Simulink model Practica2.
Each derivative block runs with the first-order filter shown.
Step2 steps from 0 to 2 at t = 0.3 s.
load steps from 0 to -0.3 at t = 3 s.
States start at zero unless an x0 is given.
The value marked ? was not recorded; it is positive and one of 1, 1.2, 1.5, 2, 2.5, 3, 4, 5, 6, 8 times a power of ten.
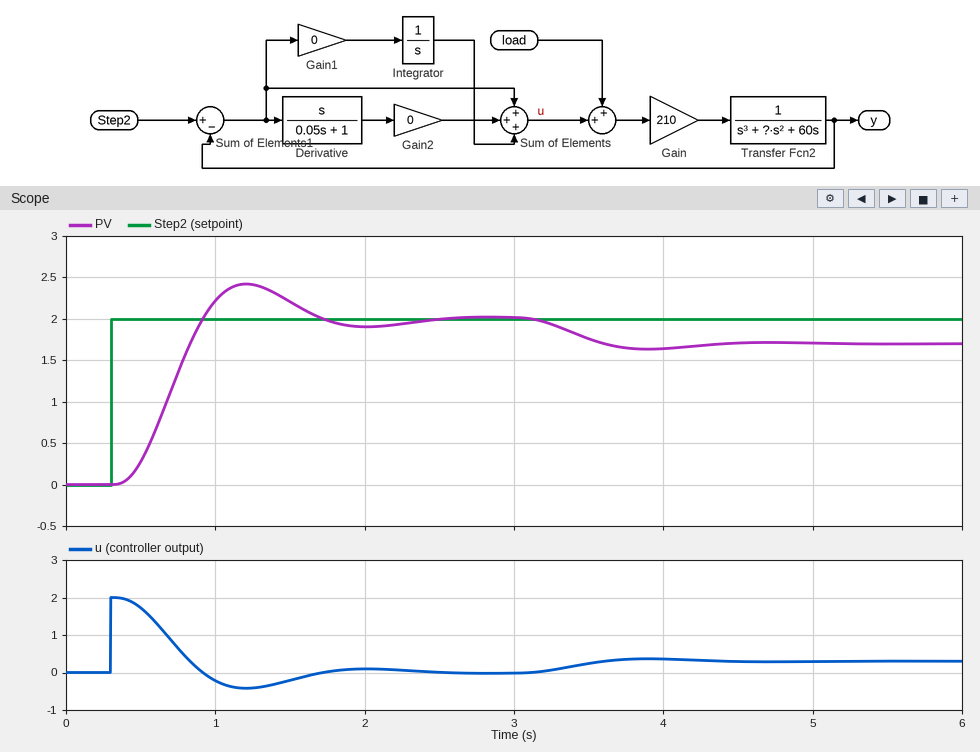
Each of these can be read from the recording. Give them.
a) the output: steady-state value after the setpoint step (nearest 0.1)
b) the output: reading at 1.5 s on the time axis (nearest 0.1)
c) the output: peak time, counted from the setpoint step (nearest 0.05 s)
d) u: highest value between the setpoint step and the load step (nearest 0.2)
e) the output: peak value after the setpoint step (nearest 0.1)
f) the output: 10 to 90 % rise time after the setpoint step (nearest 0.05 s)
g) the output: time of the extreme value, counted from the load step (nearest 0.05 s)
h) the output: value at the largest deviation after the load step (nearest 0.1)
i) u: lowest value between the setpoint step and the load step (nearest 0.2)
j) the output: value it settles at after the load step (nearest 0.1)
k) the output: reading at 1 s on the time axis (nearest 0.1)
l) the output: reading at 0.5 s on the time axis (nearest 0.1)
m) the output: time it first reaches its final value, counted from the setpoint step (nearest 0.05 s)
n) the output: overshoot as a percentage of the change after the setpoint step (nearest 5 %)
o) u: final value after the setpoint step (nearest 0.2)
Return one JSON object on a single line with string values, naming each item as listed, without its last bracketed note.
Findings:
{"the output: steady-state value after the setpoint step": "2.0", "the output: reading at 1.5 s on the time axis": "2.2", "the output: peak time, counted from the setpoint step": "0.90 s", "u: highest value between the setpoint step and the load step": "2.0", "the output: peak value after the setpoint step": "2.4", "the output: 10 to 90 % rise time after the setpoint step": "0.40 s", "the output: time of the extreme value, counted from the load step": "0.90 s", "the output: value at the largest deviation after the load step": "1.6", "u: lowest value between the setpoint step and the load step": "-0.4", "the output: value it settles at after the load step": "1.7", "the output: reading at 1 s on the time axis": "2.2", "the output: reading at 0.5 s on the time axis": "0.3", "the output: time it first reaches its final value, counted from the setpoint step": "0.60 s", "the output: overshoot as a percentage of the change after the setpoint step": "20 %", "u: final value after the setpoint step": "0.0"}
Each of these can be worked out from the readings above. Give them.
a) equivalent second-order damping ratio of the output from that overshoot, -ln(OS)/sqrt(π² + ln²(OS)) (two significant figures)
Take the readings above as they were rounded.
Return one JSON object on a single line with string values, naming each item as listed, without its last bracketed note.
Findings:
{"equivalent second-order damping ratio of the output from that overshoot, -ln(OS)/sqrt(π² + ln²(OS))": "0.46"}
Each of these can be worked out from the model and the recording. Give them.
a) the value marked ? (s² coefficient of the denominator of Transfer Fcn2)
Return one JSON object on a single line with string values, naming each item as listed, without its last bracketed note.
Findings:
{"the value marked ?": "15"}
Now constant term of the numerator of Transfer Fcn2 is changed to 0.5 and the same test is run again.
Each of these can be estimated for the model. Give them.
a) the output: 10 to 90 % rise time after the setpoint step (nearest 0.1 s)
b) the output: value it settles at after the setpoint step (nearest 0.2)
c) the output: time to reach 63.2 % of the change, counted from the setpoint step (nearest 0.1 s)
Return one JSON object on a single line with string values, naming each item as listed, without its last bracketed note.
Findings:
{"the output: 10 to 90 % rise time after the setpoint step": "0.8 s", "the output: value it settles at after the setpoint step": "2.0", "the output: time to reach 63.2 % of the change, counted from the setpoint step": "0.7 s"}
